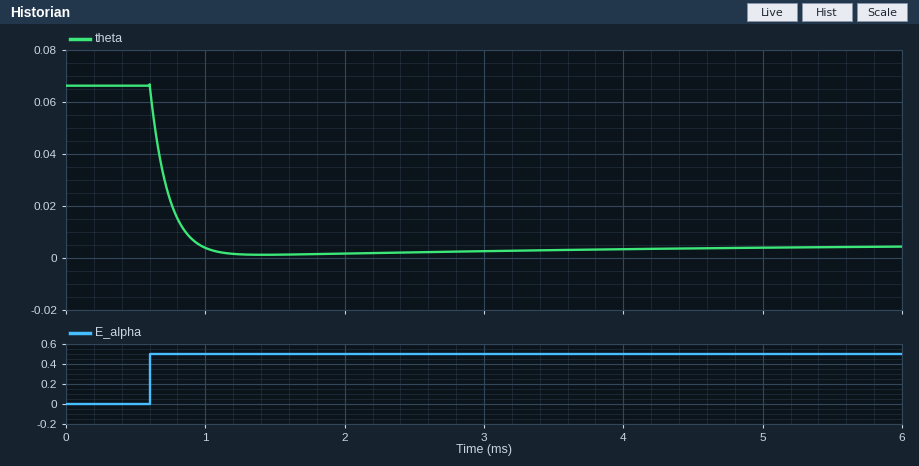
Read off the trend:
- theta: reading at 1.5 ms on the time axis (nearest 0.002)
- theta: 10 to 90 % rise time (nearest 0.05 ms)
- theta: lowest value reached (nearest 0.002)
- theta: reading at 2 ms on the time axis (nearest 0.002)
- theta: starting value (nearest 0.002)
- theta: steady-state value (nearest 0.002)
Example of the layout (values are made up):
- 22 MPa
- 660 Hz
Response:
- 0.002
- 0.25 ms
- 0.002
- 0.002
- 0.066
- 0.004
